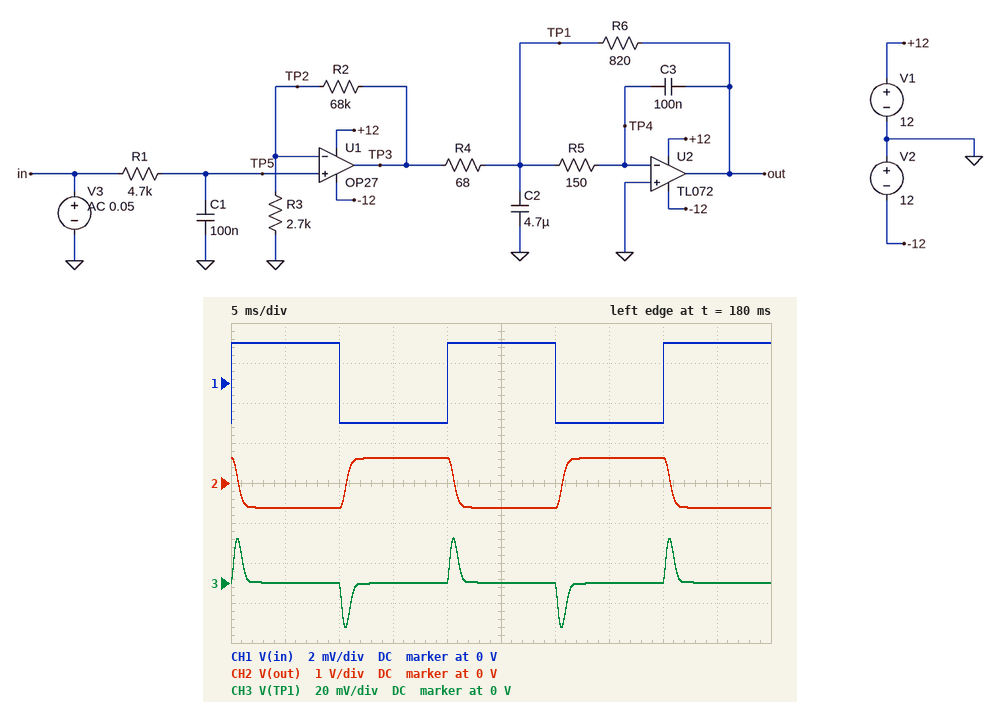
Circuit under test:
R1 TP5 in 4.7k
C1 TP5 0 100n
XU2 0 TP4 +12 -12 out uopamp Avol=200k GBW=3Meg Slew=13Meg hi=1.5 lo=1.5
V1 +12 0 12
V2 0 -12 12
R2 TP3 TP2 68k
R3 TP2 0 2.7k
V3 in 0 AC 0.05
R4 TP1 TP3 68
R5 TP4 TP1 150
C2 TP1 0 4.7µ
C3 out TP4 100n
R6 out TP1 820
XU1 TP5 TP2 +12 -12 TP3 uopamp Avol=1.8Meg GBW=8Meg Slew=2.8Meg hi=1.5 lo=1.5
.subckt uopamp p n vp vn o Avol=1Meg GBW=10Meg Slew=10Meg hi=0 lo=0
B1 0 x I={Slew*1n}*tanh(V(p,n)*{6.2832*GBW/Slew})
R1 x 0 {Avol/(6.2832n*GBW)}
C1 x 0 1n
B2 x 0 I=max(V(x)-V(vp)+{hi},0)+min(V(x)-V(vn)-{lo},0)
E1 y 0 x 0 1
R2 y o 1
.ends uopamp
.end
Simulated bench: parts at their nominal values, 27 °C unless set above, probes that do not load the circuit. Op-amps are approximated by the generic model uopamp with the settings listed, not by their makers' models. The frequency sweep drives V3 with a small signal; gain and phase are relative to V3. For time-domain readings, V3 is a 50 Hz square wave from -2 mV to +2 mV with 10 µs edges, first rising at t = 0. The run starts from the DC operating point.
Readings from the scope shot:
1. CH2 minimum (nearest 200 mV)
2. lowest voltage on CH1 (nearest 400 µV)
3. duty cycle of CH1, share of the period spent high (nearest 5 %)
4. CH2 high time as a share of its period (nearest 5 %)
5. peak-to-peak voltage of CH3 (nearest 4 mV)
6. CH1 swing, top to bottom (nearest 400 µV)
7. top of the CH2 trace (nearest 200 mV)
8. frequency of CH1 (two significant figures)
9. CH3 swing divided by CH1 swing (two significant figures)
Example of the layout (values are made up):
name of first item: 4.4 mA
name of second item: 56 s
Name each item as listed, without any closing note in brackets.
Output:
CH2 minimum: -600 mV
lowest voltage on CH1: -2.0 mV
duty cycle of CH1, share of the period spent high: 50 %
CH2 high time as a share of its period: 50 %
peak-to-peak voltage of CH3: 44 mV
CH1 swing, top to bottom: 4.0 mV
top of the CH2 trace: 600 mV
frequency of CH1: 50 Hz
CH3 swing divided by CH1 swing: 11
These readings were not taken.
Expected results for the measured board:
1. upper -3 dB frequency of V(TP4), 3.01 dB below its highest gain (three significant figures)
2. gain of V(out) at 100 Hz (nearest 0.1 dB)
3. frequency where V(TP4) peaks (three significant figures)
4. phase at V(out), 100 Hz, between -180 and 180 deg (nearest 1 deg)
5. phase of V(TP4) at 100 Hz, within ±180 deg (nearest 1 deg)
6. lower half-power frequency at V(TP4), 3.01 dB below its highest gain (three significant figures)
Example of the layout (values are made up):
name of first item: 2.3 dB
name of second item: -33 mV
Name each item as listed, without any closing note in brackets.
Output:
upper -3 dB frequency of V(TP4), 3.01 dB below its highest gain: 821 Hz
gain of V(out) at 100 Hz: 49.7 dB
frequency where V(TP4) peaks: 505 Hz
phase at V(out), 100 Hz, between -180 and 180 deg: 153 deg
phase of V(TP4) at 100 Hz, within ±180 deg: 55 deg
lower half-power frequency at V(TP4), 3.01 dB below its highest gain: 240 Hz
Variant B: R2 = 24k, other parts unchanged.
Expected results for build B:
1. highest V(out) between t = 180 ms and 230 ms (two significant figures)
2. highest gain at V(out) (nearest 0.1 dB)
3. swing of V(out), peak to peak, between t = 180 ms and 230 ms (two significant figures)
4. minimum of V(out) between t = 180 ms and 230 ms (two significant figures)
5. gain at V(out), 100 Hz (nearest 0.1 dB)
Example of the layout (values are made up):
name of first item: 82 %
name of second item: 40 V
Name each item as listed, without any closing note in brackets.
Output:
highest V(out) between t = 180 ms and 230 ms: 240 mV
highest gain at V(out): 41.5 dB
swing of V(out), peak to peak, between t = 180 ms and 230 ms: 480 mV
minimum of V(out) between t = 180 ms and 230 ms: -240 mV
gain at V(out), 100 Hz: 41.2 dB
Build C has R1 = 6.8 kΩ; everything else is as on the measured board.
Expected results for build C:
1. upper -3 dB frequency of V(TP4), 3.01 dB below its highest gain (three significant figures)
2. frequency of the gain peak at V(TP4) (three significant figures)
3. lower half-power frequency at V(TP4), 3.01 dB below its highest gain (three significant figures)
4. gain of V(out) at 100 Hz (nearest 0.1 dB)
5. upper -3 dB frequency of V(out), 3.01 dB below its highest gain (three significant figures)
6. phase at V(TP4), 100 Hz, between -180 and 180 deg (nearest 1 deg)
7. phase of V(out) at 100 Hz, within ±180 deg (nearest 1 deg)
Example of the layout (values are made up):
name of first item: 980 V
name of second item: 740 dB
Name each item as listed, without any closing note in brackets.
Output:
upper -3 dB frequency of V(TP4), 3.01 dB below its highest gain: 792 Hz
frequency of the gain peak at V(TP4): 472 Hz
lower half-power frequency at V(TP4), 3.01 dB below its highest gain: 196 Hz
gain of V(out) at 100 Hz: 49.3 dB
upper -3 dB frequency of V(out), 3.01 dB below its highest gain: 252 Hz
phase at V(TP4), 100 Hz, between -180 and 180 deg: 48 deg
phase of V(out) at 100 Hz, within ±180 deg: 147 deg
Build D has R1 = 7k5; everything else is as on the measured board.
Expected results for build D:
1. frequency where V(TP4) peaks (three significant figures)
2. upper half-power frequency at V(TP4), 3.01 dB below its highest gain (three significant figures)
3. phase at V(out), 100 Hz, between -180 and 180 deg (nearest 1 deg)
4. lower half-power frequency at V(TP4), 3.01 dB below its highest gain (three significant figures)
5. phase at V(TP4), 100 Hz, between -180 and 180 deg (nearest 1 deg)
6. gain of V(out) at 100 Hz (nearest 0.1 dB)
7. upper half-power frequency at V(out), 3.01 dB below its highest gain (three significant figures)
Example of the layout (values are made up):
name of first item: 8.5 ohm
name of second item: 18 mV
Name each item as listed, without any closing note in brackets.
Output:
frequency where V(TP4) peaks: 463 Hz
upper half-power frequency at V(TP4), 3.01 dB below its highest gain: 786 Hz
phase at V(out), 100 Hz, between -180 and 180 deg: 145 deg
lower half-power frequency at V(TP4), 3.01 dB below its highest gain: 184 Hz
phase at V(TP4), 100 Hz, between -180 and 180 deg: 46 deg
gain of V(out) at 100 Hz: 49.2 dB
upper half-power frequency at V(out), 3.01 dB below its highest gain: 226 Hz
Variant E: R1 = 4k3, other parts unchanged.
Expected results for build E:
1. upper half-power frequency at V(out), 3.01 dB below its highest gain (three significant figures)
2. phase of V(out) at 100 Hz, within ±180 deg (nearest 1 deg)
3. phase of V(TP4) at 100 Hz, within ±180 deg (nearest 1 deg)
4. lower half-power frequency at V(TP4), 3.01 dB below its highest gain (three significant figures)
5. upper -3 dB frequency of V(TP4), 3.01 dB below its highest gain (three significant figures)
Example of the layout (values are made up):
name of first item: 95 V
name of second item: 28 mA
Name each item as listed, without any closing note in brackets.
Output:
upper half-power frequency at V(out), 3.01 dB below its highest gain: 412 Hz
phase of V(out) at 100 Hz, within ±180 deg: 155 deg
phase of V(TP4) at 100 Hz, within ±180 deg: 56 deg
lower half-power frequency at V(TP4), 3.01 dB below its highest gain: 251 Hz
upper -3 dB frequency of V(TP4), 3.01 dB below its highest gain: 830 Hz
